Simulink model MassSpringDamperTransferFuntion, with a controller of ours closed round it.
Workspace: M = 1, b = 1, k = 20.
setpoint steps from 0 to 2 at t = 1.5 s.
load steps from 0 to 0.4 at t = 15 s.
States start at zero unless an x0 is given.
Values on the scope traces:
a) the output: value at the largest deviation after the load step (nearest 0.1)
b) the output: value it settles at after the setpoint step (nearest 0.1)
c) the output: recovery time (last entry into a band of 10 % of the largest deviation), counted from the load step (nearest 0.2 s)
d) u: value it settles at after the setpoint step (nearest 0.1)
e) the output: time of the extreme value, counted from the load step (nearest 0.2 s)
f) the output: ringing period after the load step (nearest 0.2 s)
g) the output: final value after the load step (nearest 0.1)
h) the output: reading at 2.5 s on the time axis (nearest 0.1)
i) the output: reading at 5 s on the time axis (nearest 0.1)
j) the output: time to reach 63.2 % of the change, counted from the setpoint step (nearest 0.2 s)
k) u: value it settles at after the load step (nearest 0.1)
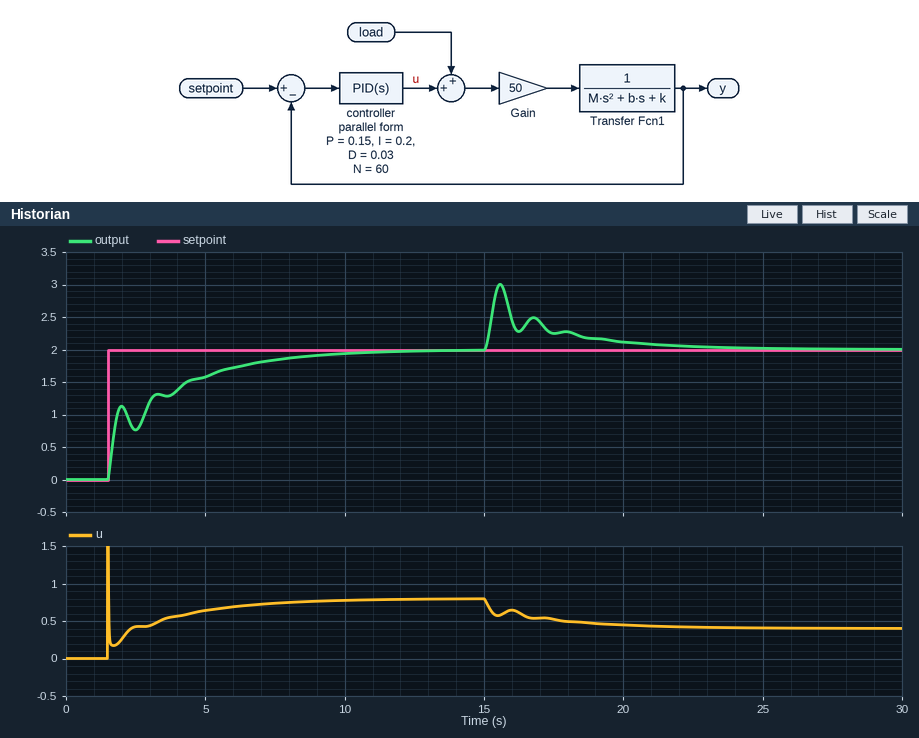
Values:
3.0
2.0
5.4 s
0.8
0.6 s
1.2 s
2.0
0.8
1.6
1.6 s
0.4
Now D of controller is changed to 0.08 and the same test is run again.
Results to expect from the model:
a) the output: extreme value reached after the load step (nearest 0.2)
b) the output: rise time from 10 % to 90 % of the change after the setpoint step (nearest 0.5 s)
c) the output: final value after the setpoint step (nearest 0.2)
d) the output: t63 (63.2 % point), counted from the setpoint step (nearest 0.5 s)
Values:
2.8
5.5 s
2.0
2.0 s
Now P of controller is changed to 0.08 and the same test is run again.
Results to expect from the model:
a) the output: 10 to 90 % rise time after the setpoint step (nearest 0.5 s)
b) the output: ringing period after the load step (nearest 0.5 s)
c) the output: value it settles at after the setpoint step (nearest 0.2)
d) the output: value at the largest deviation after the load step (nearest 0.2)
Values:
5.0 s
1.5 s
2.0
3.2
